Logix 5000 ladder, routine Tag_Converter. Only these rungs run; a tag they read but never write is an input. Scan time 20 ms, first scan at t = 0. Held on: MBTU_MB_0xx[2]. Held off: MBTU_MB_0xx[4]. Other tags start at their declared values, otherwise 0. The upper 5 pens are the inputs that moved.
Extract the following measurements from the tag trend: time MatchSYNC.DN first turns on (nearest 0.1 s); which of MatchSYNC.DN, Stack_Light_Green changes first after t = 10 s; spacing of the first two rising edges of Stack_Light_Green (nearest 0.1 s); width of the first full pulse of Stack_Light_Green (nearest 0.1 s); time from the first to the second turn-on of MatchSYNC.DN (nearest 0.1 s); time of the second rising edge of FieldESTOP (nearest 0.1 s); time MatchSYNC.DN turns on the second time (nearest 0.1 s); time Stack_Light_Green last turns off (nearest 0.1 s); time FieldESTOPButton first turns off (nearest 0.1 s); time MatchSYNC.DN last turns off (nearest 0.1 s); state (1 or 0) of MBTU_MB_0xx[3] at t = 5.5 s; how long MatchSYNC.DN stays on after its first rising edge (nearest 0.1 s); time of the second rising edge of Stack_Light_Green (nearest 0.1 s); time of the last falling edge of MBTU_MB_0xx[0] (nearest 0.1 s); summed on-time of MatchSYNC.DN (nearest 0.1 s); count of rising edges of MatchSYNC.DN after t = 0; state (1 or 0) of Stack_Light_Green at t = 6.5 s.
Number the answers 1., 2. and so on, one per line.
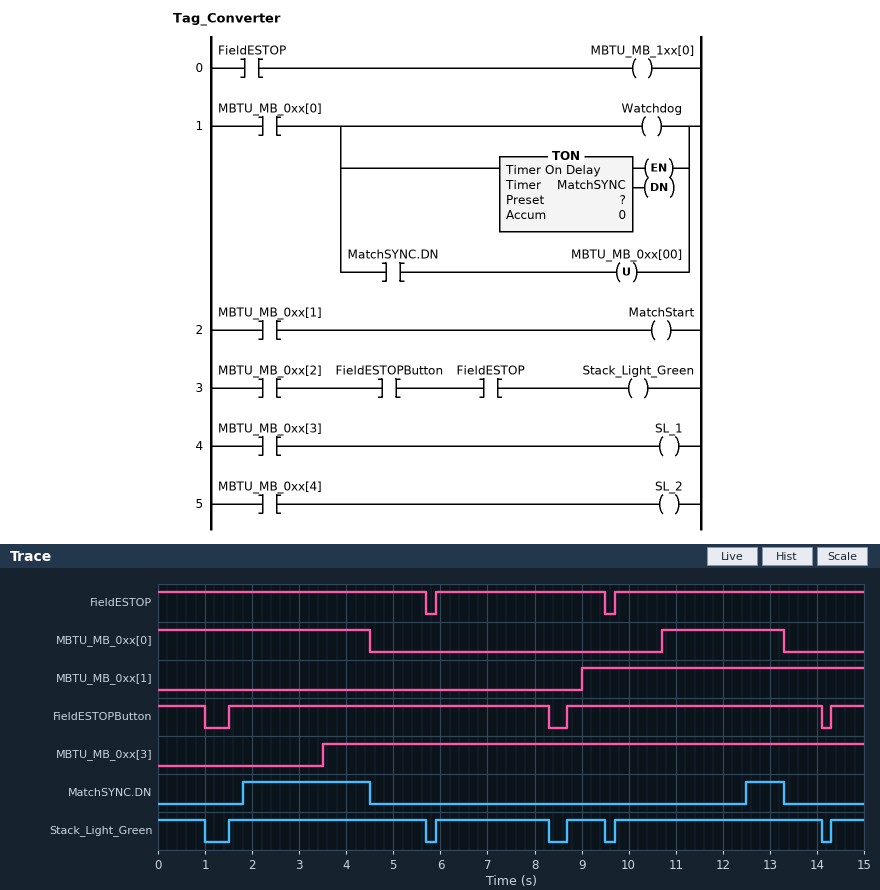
1. 1.8 s
2. MatchSYNC.DN
3. 4.4 s
4. 4.2 s
5. 10.7 s
6. 9.7 s
7. 12.5 s
8. 14.1 s
9. 1.0 s
10. 13.3 s
11. 1
12. 2.7 s
13. 5.9 s
14. 13.3 s
15. 3.5 s
16. 2
17. 1
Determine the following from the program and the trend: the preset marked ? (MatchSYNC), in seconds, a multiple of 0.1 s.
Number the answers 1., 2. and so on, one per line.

1. 1.8 s
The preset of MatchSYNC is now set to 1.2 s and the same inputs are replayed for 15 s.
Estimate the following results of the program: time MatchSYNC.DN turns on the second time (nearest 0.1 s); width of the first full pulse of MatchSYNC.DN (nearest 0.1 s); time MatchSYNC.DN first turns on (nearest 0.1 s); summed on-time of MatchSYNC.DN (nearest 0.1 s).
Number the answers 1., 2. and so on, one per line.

1. 11.9 s
2. 3.3 s
3. 1.2 s
4. 4.7 s
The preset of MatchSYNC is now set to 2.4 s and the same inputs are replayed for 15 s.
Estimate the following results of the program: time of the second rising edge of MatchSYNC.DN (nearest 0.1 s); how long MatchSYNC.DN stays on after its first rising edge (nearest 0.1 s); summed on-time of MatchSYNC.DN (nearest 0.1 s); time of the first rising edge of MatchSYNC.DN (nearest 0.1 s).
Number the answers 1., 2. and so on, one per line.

1. 13.1 s
2. 2.1 s
3. 2.3 s
4. 2.4 s
